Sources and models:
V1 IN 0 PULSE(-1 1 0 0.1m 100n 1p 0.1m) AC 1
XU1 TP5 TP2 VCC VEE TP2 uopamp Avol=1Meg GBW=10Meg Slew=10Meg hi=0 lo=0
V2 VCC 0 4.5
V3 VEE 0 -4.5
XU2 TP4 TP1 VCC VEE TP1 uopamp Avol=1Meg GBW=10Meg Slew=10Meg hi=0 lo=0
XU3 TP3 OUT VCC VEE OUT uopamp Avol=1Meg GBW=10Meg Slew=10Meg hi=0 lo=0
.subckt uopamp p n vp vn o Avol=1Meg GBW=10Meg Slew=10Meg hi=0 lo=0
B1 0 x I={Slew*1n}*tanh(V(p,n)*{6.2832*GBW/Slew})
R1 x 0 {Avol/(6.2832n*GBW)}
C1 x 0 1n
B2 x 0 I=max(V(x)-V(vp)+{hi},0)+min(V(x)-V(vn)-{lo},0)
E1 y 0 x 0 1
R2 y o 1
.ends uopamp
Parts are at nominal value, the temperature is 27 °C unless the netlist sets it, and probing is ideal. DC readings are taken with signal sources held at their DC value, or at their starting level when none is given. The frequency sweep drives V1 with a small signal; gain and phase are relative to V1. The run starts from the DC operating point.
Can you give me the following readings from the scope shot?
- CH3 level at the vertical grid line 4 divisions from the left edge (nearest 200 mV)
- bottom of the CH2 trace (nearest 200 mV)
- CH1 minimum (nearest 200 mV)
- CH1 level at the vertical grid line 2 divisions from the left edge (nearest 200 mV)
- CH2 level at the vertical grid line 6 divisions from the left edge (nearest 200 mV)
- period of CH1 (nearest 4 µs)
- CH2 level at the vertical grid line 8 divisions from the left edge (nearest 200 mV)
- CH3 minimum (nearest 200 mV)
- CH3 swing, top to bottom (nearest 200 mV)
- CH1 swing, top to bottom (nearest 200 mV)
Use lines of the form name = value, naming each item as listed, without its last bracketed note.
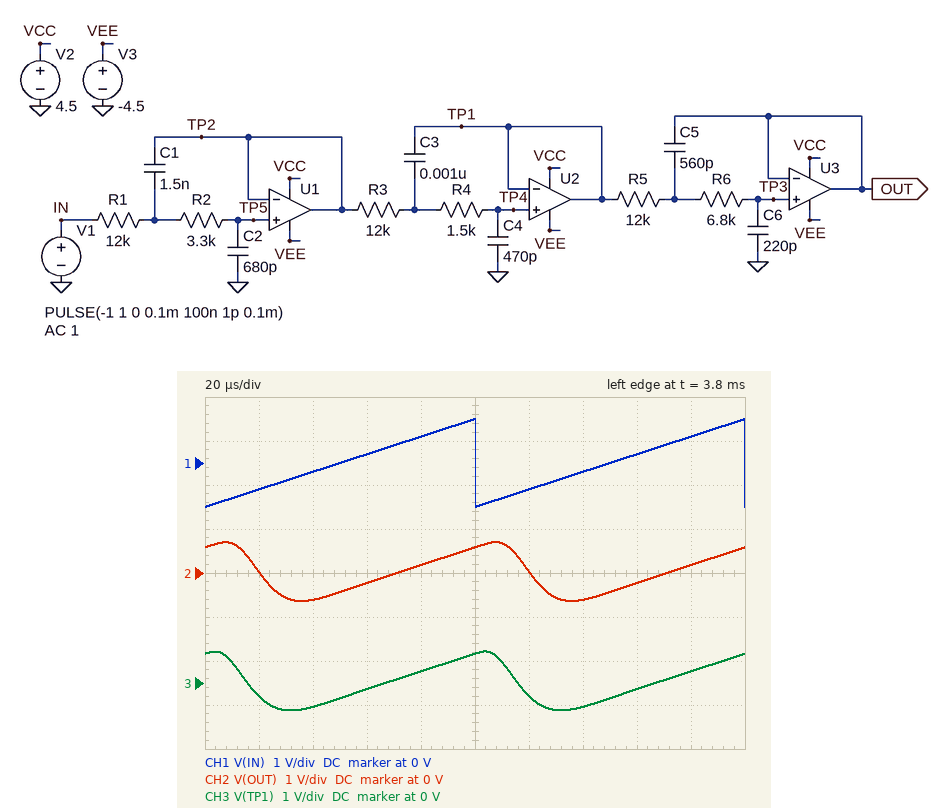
CH3 level at the vertical grid line 4 divisions from the left edge = 200 mV
bottom of the CH2 trace = -600 mV
CH1 minimum = -1.0 V
CH1 level at the vertical grid line 2 divisions from the left edge = -200 mV
CH2 level at the vertical grid line 6 divisions from the left edge = 0 V
period of CH1 = 100 µs
CH2 level at the vertical grid line 8 divisions from the left edge = -200 mV
CH3 minimum = -600 mV
CH3 swing, top to bottom = 1.4 V
CH1 swing, top to bottom = 2.0 V
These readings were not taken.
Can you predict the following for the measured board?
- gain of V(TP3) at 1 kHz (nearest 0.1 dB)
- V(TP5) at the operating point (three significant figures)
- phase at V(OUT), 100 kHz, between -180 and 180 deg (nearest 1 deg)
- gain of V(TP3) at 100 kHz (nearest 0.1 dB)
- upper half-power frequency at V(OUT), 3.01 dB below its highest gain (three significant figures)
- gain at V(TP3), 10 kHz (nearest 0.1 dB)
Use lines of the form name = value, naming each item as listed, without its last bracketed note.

gain of V(TP3) at 1 kHz = 0 dB
V(TP5) at the operating point = -1.00 V
phase at V(OUT), 100 kHz, between -180 and 180 deg = -59 deg
gain of V(TP3) at 100 kHz = -49.7 dB
upper half-power frequency at V(OUT), 3.01 dB below its highest gain = 17.7 kHz
gain at V(TP3), 10 kHz = -0.9 dB
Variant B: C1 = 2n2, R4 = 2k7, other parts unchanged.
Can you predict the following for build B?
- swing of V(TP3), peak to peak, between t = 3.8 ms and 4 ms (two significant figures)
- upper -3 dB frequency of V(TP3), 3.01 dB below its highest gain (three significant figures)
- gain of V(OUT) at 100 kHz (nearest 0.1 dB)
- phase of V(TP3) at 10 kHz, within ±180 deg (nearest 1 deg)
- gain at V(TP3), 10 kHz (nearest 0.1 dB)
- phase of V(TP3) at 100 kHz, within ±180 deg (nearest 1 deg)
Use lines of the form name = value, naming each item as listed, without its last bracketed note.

swing of V(TP3), peak to peak, between t = 3.8 ms and 4 ms = 1.4 V
upper -3 dB frequency of V(TP3), 3.01 dB below its highest gain = 19.1 kHz
gain of V(OUT) at 100 kHz = -55.9 dB
phase of V(TP3) at 10 kHz, within ±180 deg = -81 deg
gain at V(TP3), 10 kHz = -0.3 dB
phase of V(TP3) at 100 kHz, within ±180 deg = -84 deg
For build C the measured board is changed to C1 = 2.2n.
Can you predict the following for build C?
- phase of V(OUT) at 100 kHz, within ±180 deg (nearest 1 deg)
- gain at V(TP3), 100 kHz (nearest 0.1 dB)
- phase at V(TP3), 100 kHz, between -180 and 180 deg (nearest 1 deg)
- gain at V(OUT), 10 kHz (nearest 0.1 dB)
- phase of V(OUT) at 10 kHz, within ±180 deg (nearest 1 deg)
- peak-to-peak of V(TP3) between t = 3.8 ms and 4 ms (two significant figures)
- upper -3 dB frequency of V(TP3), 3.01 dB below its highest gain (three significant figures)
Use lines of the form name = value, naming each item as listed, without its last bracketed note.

phase of V(OUT) at 100 kHz, within ±180 deg = -66 deg
gain at V(TP3), 100 kHz = -52.8 dB
phase at V(TP3), 100 kHz, between -180 and 180 deg = -65 deg
gain at V(OUT), 10 kHz = -0.4 dB
phase of V(OUT) at 10 kHz, within ±180 deg = -78 deg
peak-to-peak of V(TP3) between t = 3.8 ms and 4 ms = 1.4 V
upper -3 dB frequency of V(TP3), 3.01 dB below its highest gain = 18.8 kHz
